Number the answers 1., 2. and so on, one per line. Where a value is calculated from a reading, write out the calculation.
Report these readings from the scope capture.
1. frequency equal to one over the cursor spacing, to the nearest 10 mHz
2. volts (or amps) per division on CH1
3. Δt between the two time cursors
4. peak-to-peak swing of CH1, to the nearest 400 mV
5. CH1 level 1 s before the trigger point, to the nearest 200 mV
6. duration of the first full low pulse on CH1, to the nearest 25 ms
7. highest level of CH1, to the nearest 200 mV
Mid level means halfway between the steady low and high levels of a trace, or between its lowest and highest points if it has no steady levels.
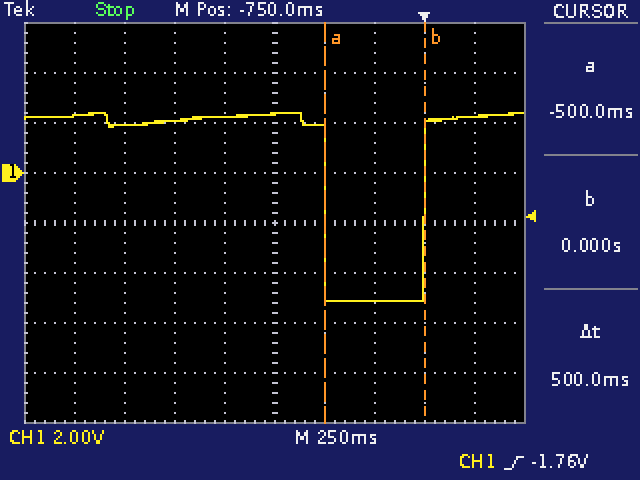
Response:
1. 1 / 500 ms ≈ 2.00 Hz
2. 2 V
3. 500 ms
4. 7.6 V
5. 2.2 V
6. 500 ms
7. 2.4 V
